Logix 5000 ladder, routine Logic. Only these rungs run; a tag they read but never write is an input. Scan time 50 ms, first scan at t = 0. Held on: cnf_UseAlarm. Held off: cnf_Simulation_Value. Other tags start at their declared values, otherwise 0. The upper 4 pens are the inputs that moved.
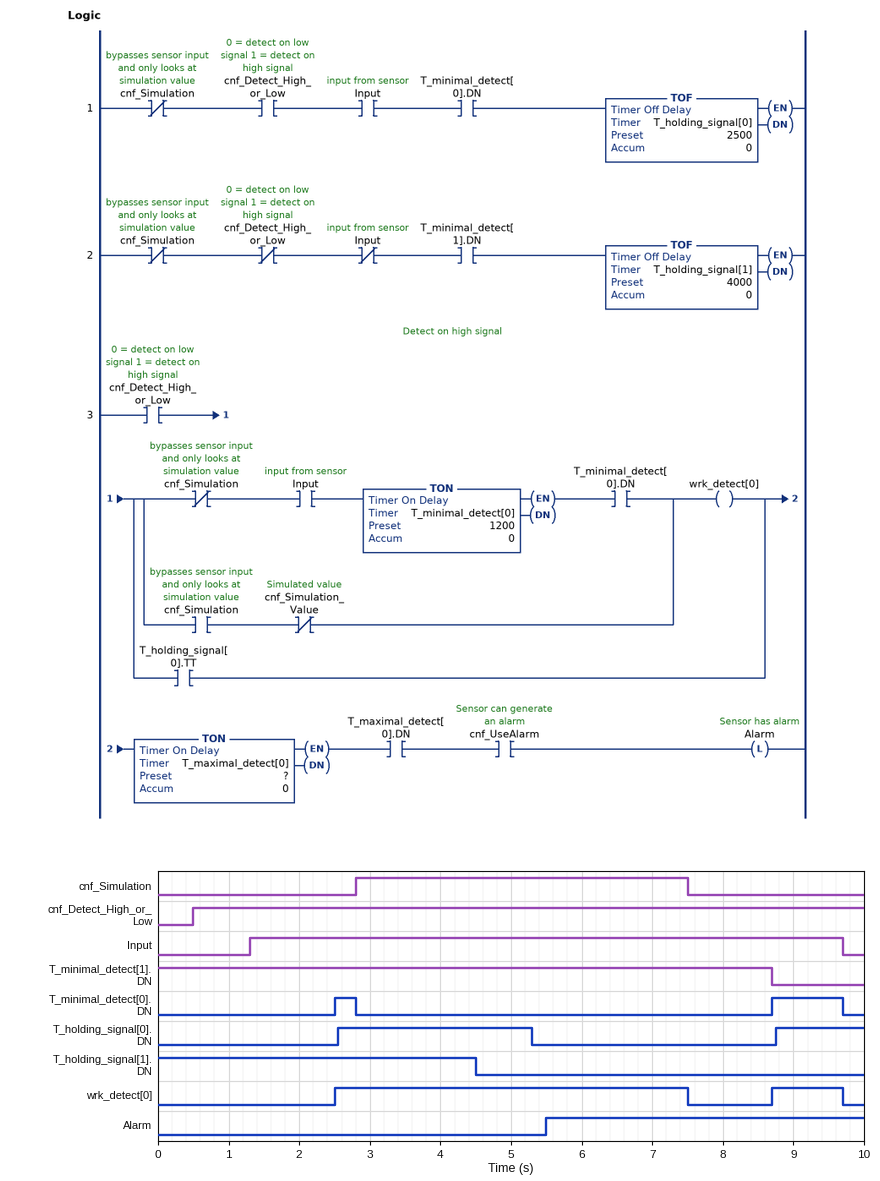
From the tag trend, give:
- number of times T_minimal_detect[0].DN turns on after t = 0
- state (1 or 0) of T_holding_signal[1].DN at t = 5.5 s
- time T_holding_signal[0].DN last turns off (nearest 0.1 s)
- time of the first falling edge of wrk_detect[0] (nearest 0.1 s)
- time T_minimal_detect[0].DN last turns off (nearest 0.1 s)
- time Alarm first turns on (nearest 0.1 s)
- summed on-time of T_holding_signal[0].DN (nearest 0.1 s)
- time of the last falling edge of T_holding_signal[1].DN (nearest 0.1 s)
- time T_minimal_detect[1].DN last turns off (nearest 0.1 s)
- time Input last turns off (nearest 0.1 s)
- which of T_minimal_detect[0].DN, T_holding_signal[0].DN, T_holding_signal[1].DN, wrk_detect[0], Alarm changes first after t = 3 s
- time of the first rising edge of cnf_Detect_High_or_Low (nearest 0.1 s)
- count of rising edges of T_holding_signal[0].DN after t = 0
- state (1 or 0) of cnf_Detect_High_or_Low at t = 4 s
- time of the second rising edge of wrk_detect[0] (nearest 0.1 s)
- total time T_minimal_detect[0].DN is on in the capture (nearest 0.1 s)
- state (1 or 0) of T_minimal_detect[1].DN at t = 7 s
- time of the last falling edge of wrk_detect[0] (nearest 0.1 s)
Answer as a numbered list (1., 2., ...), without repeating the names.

1. 2
2. 0
3. 5.3 s
4. 7.5 s
5. 9.7 s
6. 5.5 s
7. 4.0 s
8. 4.5 s
9. 8.7 s
10. 9.7 s
11. T_holding_signal[1].DN
12. 0.5 s
13. 2
14. 1
15. 8.7 s
16. 1.3 s
17. 1
18. 9.7 s
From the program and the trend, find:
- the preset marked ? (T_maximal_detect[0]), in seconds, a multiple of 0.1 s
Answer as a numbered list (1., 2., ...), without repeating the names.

1. 3.0 s
